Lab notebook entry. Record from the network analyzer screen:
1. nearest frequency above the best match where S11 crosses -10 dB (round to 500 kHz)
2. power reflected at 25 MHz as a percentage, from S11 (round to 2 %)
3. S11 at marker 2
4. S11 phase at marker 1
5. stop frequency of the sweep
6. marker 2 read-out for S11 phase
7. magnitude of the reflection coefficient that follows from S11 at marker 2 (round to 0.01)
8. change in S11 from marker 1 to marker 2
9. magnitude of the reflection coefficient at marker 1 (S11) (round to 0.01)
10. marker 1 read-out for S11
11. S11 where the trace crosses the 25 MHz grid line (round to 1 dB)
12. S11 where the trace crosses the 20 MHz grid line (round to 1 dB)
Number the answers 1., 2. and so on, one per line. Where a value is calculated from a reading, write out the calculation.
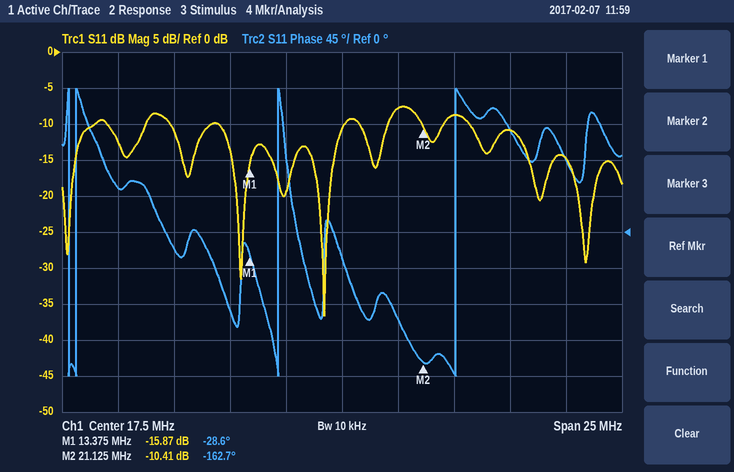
1. 17.5 MHz
2. 10^(-11/10) ≈ 8 %
3. -10.41 dB
4. -28.6°
5. 30 MHz
6. -162.7°
7. 10^(-10.41/20) ≈ 0.30
8. -10.41 − (-15.87) = 5.46 dB
9. 10^(-15.87/20) ≈ 0.16
10. -15.87 dB
11. -11 dB
12. -8 dB
